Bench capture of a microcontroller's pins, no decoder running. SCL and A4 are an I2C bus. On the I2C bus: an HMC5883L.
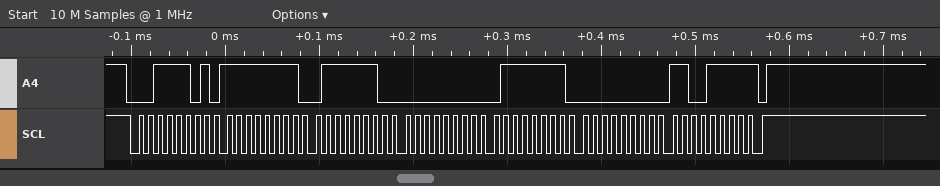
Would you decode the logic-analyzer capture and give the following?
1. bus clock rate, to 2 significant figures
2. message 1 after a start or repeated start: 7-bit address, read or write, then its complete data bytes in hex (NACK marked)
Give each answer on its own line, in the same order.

100 kHz
0x1E read: FF 7E 00 7F 00 CF NACK
